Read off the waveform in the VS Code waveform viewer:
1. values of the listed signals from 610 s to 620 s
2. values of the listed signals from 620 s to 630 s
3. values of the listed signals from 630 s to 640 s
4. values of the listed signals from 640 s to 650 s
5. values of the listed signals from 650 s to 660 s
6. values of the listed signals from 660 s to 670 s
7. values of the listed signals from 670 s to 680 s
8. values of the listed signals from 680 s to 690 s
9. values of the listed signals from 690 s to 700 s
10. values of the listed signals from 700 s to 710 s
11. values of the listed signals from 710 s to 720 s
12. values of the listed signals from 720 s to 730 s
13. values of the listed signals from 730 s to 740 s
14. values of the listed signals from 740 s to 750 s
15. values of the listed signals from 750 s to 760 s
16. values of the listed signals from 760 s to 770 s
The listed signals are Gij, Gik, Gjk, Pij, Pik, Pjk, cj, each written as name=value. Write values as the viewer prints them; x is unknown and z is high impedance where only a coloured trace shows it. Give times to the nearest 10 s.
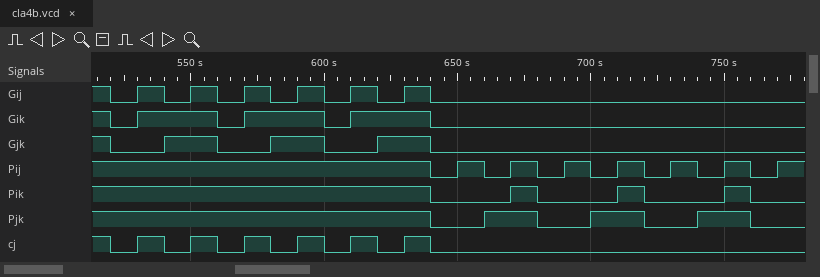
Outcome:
Gij=1, Gik=1, Gjk=0, Pij=1, Pik=1, Pjk=1, cj=1
Gij=0, Gik=1, Gjk=1, Pij=1, Pik=1, Pjk=1, cj=0
Gij=1, Gik=1, Gjk=1, Pij=1, Pik=1, Pjk=1, cj=1
Gij=0, Gik=0, Gjk=0, Pij=0, Pik=0, Pjk=0, cj=0
Gij=0, Gik=0, Gjk=0, Pij=1, Pik=0, Pjk=0, cj=0
Gij=0, Gik=0, Gjk=0, Pij=0, Pik=0, Pjk=1, cj=0
Gij=0, Gik=0, Gjk=0, Pij=1, Pik=1, Pjk=1, cj=0
Gij=0, Gik=0, Gjk=0, Pij=0, Pik=0, Pjk=0, cj=0
Gij=0, Gik=0, Gjk=0, Pij=1, Pik=0, Pjk=0, cj=0
Gij=0, Gik=0, Gjk=0, Pij=0, Pik=0, Pjk=1, cj=0
Gij=0, Gik=0, Gjk=0, Pij=1, Pik=1, Pjk=1, cj=0
Gij=0, Gik=0, Gjk=0, Pij=0, Pik=0, Pjk=0, cj=0
Gij=0, Gik=0, Gjk=0, Pij=1, Pik=0, Pjk=0, cj=0
Gij=0, Gik=0, Gjk=0, Pij=0, Pik=0, Pjk=1, cj=0
Gij=0, Gik=0, Gjk=0, Pij=1, Pik=1, Pjk=1, cj=0
Gij=0, Gik=0, Gjk=0, Pij=0, Pik=0, Pjk=0, cj=0
